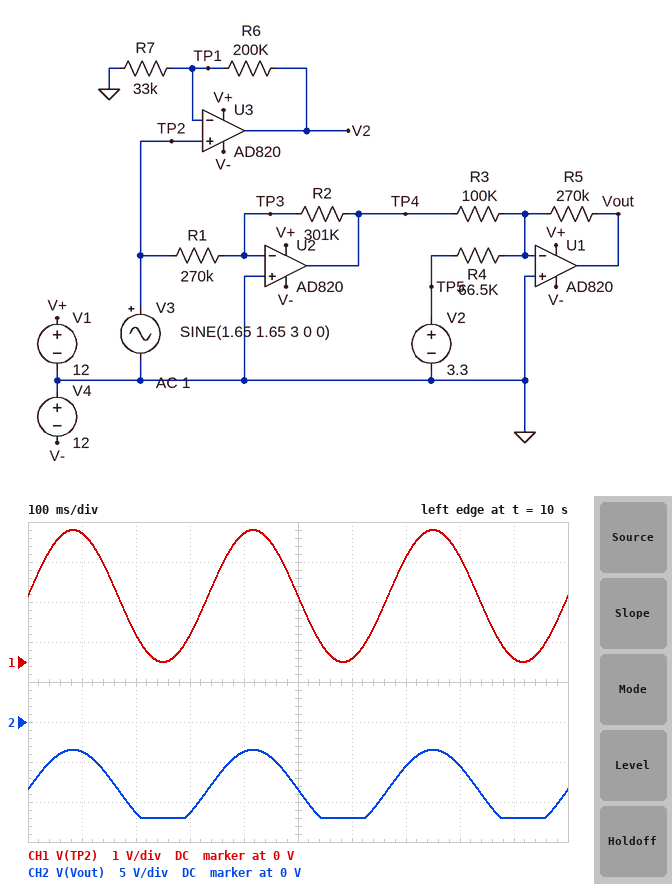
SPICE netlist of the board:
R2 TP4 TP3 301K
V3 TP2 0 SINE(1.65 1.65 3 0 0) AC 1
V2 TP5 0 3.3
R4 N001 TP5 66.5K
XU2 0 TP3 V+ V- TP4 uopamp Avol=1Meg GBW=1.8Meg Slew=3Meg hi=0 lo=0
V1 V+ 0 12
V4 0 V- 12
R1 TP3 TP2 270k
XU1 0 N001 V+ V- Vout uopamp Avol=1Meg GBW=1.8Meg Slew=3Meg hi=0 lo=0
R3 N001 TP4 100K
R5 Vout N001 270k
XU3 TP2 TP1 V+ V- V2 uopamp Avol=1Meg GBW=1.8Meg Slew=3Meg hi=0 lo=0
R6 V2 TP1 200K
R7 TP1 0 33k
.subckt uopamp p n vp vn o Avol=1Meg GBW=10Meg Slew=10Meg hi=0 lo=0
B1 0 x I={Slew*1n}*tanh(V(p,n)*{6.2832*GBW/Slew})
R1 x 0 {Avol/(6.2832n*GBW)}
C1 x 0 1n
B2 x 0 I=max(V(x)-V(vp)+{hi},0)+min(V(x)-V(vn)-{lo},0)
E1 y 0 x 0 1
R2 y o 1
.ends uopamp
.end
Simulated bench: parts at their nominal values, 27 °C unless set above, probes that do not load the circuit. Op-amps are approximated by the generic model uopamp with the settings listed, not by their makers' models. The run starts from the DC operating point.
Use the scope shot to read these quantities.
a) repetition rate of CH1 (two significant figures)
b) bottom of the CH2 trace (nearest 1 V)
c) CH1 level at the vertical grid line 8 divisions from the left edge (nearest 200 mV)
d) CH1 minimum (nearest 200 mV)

3.0 Hz
-12 V
2.6 V
0 V
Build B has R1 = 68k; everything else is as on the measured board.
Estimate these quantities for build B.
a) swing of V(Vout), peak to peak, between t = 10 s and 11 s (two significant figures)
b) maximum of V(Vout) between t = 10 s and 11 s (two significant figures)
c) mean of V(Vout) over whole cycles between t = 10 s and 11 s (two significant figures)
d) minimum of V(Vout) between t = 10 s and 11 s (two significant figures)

24 V
12 V
2.7 V
-12 V
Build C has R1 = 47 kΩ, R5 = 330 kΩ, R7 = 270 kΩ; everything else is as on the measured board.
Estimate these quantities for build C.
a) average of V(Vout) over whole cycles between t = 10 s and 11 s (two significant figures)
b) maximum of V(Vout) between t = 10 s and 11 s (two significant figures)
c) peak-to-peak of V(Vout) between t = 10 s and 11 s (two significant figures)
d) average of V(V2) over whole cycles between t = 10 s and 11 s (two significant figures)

4.4 V
12 V
24 V
2.9 V
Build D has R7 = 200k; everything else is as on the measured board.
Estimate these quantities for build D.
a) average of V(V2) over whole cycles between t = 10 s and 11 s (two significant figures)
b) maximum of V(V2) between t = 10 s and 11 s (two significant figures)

3.3 V
6.6 V
